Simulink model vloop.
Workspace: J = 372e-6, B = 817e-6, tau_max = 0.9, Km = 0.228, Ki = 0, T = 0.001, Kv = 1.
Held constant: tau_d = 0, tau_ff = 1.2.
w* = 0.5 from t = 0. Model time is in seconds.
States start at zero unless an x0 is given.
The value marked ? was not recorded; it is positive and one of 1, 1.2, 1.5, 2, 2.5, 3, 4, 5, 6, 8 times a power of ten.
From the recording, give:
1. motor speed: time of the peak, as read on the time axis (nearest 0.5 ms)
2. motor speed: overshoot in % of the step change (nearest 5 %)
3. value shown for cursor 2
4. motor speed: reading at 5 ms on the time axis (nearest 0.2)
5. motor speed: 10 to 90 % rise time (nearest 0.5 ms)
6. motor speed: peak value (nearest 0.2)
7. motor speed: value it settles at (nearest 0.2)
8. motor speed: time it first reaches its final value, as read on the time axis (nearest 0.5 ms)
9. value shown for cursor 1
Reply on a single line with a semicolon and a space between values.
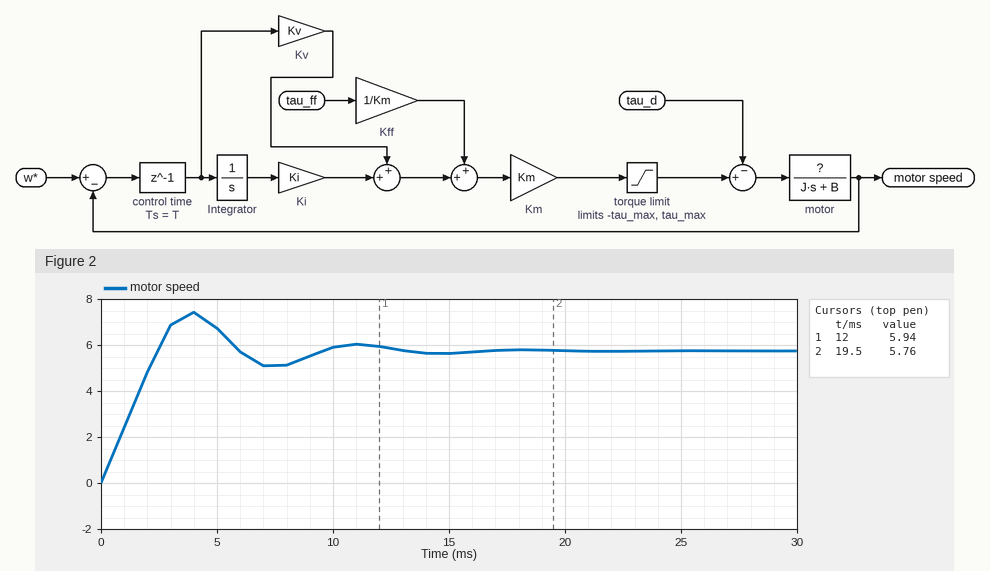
4.0 ms; 30 %; 5.76; 6.8; 2.0 ms; 7.4; 5.8; 2.5 ms; 5.94
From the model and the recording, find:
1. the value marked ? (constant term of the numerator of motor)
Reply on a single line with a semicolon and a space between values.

1
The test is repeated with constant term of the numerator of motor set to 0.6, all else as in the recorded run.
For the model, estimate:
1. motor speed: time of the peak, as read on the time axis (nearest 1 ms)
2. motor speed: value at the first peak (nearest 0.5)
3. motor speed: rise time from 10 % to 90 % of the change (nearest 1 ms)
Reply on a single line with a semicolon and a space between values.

6 ms; 6.0; 3 ms
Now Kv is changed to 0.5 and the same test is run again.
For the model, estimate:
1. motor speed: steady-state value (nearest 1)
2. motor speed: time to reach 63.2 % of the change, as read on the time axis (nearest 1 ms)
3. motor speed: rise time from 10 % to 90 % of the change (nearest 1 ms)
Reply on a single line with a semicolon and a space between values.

11; 3 ms; 4 ms
